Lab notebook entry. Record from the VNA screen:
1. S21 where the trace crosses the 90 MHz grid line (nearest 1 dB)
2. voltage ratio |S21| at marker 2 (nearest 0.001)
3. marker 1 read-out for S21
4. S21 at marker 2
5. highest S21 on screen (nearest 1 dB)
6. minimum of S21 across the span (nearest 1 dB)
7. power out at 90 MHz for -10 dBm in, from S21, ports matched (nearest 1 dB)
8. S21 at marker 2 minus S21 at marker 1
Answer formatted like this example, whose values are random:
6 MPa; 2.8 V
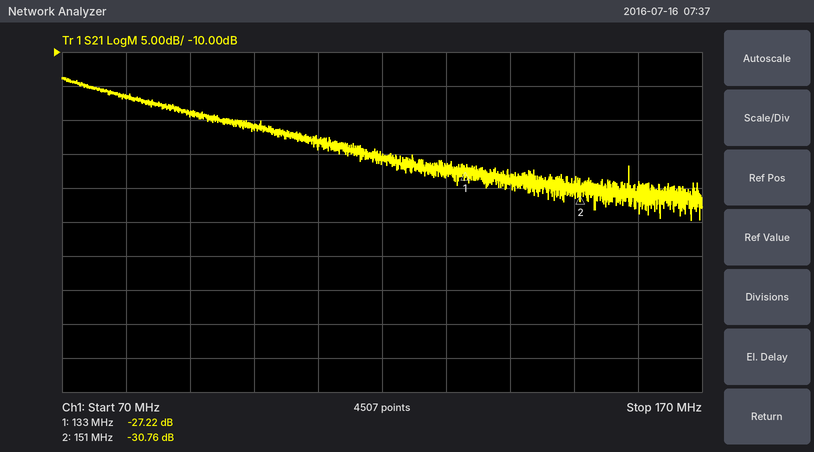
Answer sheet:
-19 dB; 0.029; -27.22 dB; -30.76 dB; -14 dB; -35 dB; -29 dBm; -3.54 dB
